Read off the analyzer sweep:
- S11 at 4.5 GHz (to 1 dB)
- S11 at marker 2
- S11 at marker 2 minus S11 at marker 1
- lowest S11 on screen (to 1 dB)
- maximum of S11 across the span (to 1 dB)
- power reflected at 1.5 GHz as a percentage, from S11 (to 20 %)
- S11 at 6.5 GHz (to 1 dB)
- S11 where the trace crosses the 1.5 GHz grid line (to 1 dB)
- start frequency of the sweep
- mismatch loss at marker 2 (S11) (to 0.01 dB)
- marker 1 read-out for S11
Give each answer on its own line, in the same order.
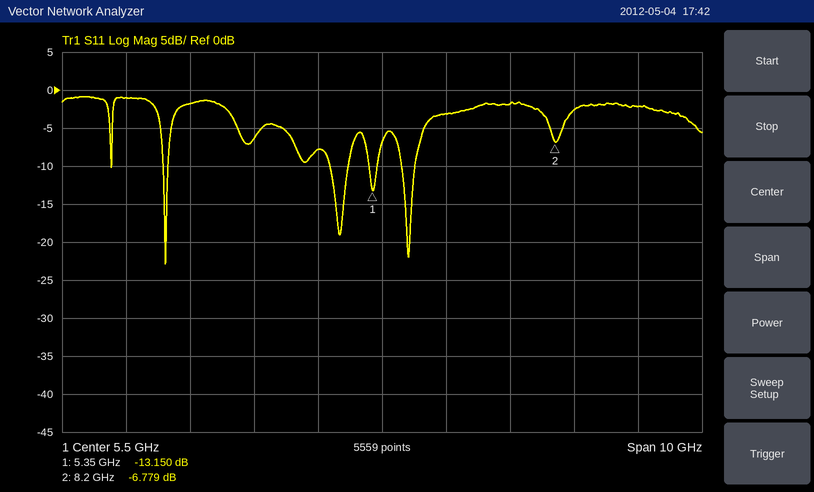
-8 dB
-6.779 dB
6.371 dB
-23 dB
-1 dB
80 %
-3 dB
-1 dB
500 MHz
1.02 dB
-13.150 dB
